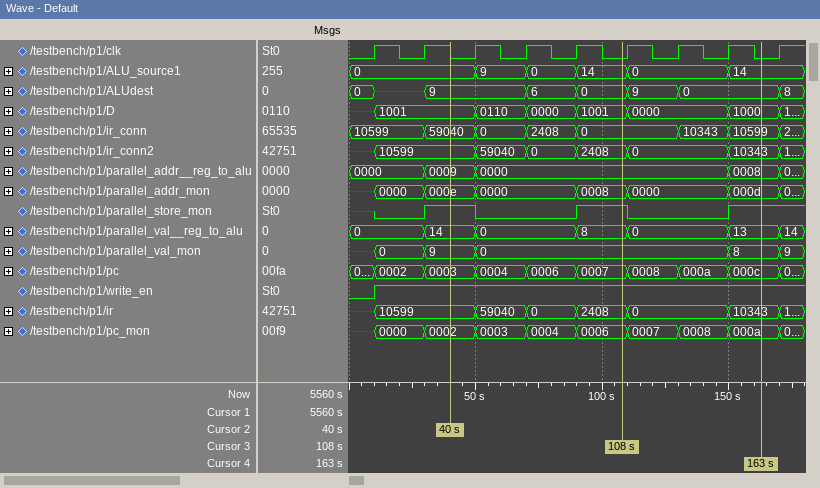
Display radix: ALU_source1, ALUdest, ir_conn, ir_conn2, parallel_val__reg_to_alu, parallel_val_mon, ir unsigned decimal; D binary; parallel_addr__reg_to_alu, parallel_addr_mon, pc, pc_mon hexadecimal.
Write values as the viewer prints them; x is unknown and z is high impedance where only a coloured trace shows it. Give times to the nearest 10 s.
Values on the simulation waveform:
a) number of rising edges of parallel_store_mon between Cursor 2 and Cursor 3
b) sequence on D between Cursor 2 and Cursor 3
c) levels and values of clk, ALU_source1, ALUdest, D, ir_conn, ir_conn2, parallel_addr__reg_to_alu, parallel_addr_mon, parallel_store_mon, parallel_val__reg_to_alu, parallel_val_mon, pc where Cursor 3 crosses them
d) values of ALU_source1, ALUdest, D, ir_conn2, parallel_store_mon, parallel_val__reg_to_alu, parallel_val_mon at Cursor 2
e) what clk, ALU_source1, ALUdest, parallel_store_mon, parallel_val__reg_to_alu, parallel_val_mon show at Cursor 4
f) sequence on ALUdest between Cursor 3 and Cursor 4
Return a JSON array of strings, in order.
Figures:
["1", "1001, 0110, 0000, 1001", "clk=0, ALU_source1=14, ALUdest=0, D=1001, ir_conn=0, ir_conn2=2408, parallel_addr__reg_to_alu=0000, parallel_addr_mon=0008, parallel_store_mon=1, parallel_val__reg_to_alu=8, parallel_val_mon=0, pc=0007", "ALU_source1=0, ALUdest=9, D=1001, ir_conn2=10599, parallel_store_mon=1, parallel_val__reg_to_alu=14, parallel_val_mon=9", "clk=0, ALU_source1=14, ALUdest=0, parallel_store_mon=1, parallel_val__reg_to_alu=13, parallel_val_mon=8", "0, 9, 0"]
